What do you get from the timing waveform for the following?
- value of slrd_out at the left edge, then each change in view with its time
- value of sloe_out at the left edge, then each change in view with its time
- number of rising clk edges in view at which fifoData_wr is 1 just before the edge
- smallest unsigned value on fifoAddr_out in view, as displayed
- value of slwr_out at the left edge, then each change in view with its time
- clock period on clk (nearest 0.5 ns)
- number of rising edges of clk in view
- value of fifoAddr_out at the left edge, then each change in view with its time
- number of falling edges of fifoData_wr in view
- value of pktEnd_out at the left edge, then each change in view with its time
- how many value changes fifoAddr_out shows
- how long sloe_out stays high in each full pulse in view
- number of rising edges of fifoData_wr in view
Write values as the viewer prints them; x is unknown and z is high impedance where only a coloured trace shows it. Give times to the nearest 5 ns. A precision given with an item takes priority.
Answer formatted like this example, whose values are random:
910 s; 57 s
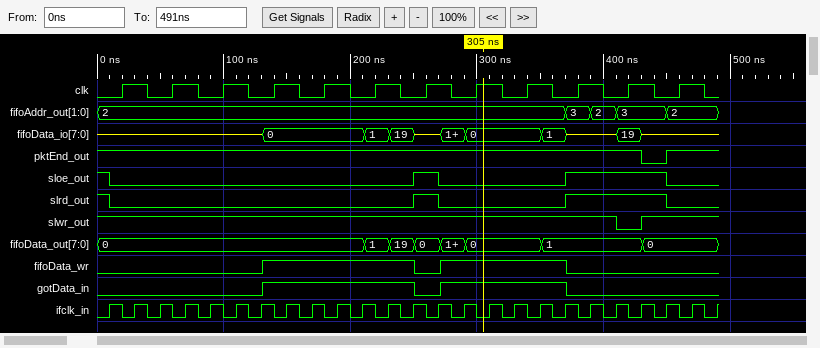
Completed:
1, 0 at 10 ns, 1 at 250 ns, 0 at 270 ns, 1 at 370 ns, 0 at 450 ns; 1, 0 at 10 ns, 1 at 250 ns, 0 at 270 ns, 1 at 370 ns, 0 at 450 ns; 5; 2; 1, 0 at 410 ns, 1 at 430 ns; 40 ns; 12; 2, 3 at 370 ns, 2 at 390 ns, 3 at 410 ns, 2 at 450 ns; 2; 1, 0 at 430 ns, 1 at 450 ns; 4; 20 ns, 80 ns; 2
